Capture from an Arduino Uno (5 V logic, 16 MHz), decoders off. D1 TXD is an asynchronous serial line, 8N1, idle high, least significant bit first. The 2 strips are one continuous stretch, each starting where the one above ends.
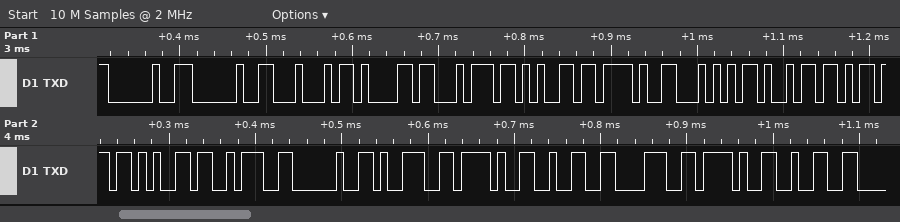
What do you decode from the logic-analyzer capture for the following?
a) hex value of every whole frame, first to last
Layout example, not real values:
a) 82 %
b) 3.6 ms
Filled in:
a) 20 20 44 61 74 65 2F 54 69 6D 65 3A 20 39 2F 32 38 2F 32
